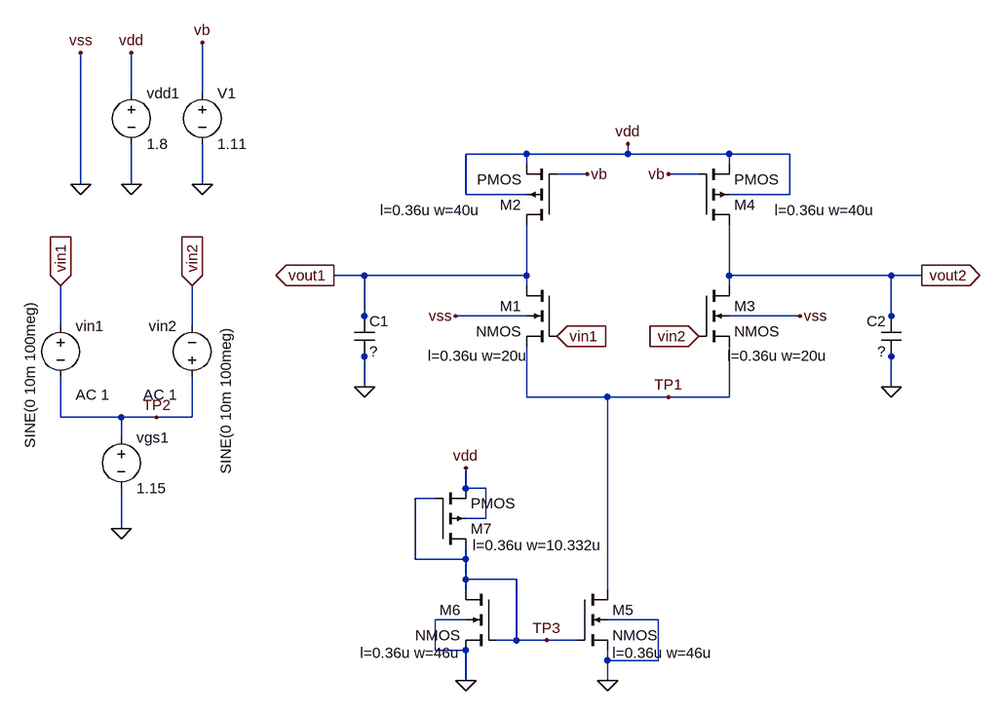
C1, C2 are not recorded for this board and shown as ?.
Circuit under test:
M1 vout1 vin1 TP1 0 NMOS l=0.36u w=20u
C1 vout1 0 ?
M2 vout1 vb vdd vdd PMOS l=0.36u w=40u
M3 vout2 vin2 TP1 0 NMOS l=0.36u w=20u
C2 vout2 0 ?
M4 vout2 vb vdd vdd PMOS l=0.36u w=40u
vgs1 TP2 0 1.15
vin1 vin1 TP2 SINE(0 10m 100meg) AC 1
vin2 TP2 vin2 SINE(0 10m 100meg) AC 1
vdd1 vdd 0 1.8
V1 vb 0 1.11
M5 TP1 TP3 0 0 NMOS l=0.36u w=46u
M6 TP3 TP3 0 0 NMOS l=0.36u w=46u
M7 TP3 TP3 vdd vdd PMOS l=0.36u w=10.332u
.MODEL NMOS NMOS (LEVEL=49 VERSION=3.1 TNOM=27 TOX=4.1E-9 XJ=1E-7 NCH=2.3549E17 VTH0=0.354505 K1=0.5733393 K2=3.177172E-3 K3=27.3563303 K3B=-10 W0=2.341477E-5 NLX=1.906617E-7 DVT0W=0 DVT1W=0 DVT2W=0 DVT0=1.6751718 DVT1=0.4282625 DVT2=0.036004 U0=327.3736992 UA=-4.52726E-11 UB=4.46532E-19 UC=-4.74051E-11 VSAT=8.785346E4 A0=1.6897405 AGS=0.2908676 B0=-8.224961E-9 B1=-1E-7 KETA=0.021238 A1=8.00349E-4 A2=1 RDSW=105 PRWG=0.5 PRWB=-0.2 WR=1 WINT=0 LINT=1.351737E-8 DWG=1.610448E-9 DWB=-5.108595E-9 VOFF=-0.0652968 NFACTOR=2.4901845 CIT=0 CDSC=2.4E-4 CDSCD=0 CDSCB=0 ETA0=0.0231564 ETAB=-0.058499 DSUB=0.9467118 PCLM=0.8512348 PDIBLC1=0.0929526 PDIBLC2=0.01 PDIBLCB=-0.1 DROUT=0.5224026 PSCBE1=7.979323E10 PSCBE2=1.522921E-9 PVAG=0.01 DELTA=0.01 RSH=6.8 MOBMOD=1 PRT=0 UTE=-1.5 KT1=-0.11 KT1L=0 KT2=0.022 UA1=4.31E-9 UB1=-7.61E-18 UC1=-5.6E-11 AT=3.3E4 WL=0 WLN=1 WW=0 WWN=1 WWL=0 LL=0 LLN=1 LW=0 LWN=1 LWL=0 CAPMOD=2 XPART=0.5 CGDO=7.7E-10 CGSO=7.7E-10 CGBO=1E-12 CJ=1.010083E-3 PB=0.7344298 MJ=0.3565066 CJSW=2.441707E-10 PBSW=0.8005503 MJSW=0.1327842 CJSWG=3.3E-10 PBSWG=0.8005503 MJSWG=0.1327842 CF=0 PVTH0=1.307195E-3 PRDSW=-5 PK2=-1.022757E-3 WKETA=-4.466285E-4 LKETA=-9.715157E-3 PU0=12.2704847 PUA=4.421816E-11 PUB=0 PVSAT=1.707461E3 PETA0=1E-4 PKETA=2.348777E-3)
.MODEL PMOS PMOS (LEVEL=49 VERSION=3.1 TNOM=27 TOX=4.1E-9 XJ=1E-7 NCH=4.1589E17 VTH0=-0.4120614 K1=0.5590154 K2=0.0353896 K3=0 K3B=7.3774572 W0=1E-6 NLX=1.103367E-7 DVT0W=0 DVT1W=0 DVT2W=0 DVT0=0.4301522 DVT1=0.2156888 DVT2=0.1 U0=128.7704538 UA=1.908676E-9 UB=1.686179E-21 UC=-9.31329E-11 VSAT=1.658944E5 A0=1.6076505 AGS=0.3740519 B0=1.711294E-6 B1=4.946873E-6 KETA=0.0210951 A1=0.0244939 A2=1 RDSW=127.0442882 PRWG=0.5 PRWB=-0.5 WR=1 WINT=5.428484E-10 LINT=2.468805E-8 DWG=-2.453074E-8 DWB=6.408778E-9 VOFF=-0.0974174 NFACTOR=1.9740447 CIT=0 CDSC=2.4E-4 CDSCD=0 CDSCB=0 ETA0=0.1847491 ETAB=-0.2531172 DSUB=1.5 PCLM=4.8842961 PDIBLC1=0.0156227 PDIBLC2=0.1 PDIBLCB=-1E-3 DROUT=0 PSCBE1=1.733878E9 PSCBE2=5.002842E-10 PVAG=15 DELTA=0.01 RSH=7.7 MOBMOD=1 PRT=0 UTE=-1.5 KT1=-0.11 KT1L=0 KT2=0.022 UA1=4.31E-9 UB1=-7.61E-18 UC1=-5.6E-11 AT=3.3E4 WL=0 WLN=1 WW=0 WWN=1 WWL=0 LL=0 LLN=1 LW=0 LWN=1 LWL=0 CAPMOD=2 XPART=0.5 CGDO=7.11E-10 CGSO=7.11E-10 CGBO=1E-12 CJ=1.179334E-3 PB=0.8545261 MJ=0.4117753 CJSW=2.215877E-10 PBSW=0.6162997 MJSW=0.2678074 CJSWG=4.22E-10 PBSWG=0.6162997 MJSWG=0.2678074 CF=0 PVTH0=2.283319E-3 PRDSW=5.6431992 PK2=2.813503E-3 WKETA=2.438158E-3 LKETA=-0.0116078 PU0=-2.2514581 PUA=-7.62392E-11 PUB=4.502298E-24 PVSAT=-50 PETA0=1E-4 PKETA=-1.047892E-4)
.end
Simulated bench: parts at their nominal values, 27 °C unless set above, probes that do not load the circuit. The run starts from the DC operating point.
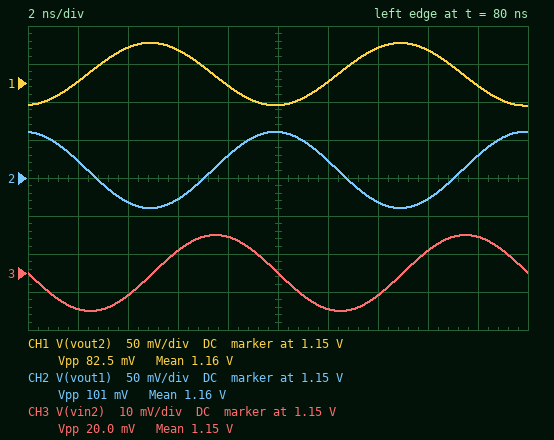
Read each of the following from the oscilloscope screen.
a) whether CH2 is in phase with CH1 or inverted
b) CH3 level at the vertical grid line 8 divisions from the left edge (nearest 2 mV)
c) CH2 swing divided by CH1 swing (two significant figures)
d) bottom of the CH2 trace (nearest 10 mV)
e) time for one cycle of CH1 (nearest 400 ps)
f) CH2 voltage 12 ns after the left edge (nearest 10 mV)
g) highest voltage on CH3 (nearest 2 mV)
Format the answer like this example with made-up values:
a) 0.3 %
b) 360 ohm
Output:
a) inverted
b) 1.156 V
c) 1.2
d) 1.11 V
e) 10.0 ns
f) 1.17 V
g) 1.160 V
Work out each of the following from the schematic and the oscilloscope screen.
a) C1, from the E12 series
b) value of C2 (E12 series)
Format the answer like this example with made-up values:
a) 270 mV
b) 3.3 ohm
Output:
a) 680 fF
b) 820 fF
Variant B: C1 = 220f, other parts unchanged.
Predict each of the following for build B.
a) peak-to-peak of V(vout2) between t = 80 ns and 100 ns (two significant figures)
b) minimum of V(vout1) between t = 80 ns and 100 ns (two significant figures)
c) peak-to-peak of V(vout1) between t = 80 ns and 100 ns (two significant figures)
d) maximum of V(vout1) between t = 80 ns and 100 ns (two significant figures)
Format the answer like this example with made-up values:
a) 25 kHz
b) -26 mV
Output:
a) 82 mV
b) 1.0 V
c) 270 mV
d) 1.3 V
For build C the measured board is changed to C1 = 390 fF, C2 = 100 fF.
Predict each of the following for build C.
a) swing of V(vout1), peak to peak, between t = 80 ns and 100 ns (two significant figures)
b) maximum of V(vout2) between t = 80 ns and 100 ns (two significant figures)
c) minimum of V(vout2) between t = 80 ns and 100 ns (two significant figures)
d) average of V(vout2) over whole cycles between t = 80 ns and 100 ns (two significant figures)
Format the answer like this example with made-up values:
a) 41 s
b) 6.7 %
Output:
a) 160 mV
b) 1.4 V
c) 950 mV
d) 1.2 V
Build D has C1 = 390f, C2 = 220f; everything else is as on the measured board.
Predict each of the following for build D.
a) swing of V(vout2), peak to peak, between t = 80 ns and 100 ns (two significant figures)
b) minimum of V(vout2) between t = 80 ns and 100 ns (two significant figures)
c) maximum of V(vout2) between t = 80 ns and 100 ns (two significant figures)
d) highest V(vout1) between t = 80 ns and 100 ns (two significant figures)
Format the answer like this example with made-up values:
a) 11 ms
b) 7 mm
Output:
a) 250 mV
b) 1.0 V
c) 1.3 V
d) 1.2 V
